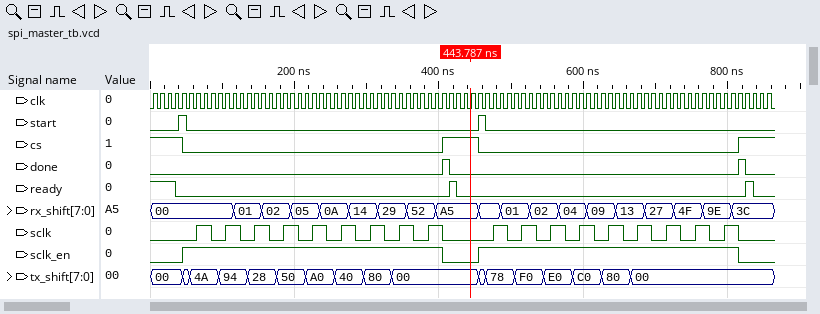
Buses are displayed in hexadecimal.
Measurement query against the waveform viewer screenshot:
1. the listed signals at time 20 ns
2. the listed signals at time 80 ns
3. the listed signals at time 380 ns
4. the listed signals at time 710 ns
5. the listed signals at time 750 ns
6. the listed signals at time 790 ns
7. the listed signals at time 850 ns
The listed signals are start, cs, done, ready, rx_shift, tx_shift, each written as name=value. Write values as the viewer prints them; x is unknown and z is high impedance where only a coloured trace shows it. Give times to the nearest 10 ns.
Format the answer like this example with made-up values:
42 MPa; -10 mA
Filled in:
start=0, cs=1, done=0, ready=1, rx_shift=00, tx_shift=00; start=0, cs=0, done=0, ready=0, rx_shift=00, tx_shift=4A; start=0, cs=0, done=0, ready=0, rx_shift=52, tx_shift=00; start=0, cs=0, done=0, ready=0, rx_shift=27, tx_shift=00; start=0, cs=0, done=0, ready=0, rx_shift=4F, tx_shift=00; start=0, cs=0, done=0, ready=0, rx_shift=9E, tx_shift=00; start=0, cs=1, done=0, ready=0, rx_shift=3C, tx_shift=00
